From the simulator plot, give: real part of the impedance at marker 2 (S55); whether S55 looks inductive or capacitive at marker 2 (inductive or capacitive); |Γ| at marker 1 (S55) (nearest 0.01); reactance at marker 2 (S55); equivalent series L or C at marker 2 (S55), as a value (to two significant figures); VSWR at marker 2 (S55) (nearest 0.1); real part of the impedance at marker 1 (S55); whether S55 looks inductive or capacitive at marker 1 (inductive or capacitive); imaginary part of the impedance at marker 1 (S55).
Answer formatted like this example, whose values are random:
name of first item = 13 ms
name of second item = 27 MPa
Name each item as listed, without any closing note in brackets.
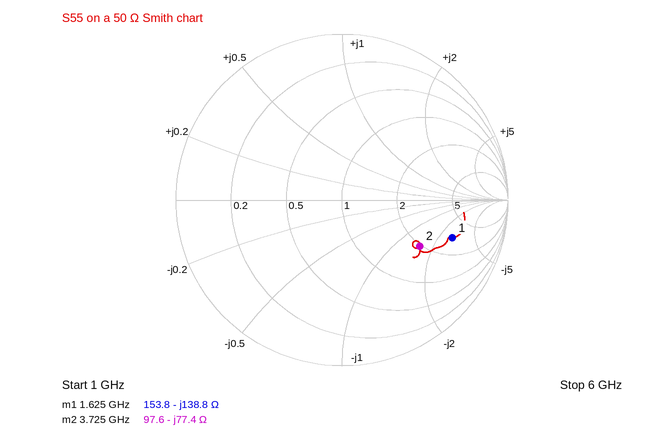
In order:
real part of the impedance at marker 2 = 97.6 Ω
whether S55 looks inductive or capacitive at marker 2 = capacitive
|Γ| at marker 1 (S55) = 0.70
reactance at marker 2 = -77.4 Ω
equivalent series L or C at marker 2 (S55), as a value = 550 fF
VSWR at marker 2 (S55) = 3.4
real part of the impedance at marker 1 = 153.8 Ω
whether S55 looks inductive or capacitive at marker 1 = capacitive
imaginary part of the impedance at marker 1 = -138.8 Ω
